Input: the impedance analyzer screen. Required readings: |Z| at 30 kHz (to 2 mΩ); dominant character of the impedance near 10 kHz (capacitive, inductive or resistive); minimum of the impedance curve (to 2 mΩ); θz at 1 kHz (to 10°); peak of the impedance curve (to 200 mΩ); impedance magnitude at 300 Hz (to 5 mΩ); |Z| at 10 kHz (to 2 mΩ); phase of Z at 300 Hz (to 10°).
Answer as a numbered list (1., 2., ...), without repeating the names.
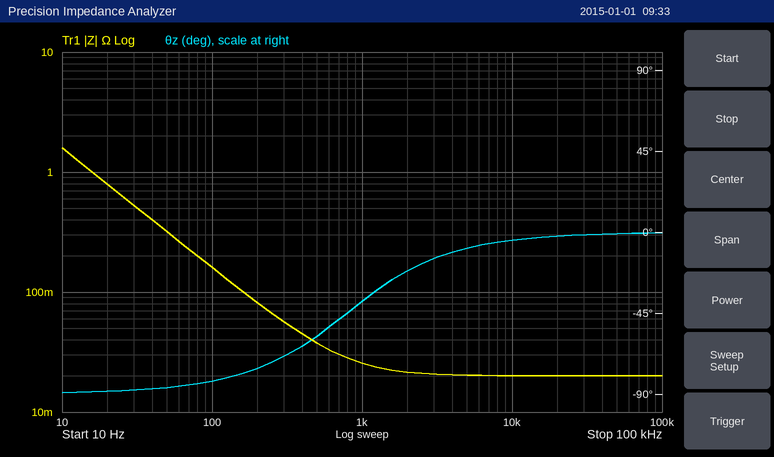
1. 20 mΩ
2. resistive
3. 20 mΩ
4. -40°
5. 1.6 Ω
6. 55 mΩ
7. 20 mΩ
8. -70°
